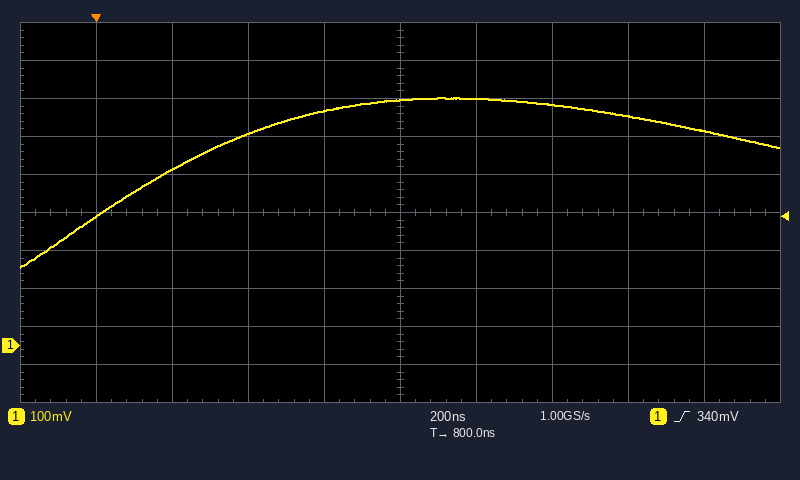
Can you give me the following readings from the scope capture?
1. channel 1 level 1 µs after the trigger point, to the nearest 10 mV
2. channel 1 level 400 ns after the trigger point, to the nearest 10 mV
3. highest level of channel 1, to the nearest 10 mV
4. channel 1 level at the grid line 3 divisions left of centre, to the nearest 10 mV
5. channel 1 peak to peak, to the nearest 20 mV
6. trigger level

650 mV
560 mV
650 mV
460 mV
440 mV
340 mV
